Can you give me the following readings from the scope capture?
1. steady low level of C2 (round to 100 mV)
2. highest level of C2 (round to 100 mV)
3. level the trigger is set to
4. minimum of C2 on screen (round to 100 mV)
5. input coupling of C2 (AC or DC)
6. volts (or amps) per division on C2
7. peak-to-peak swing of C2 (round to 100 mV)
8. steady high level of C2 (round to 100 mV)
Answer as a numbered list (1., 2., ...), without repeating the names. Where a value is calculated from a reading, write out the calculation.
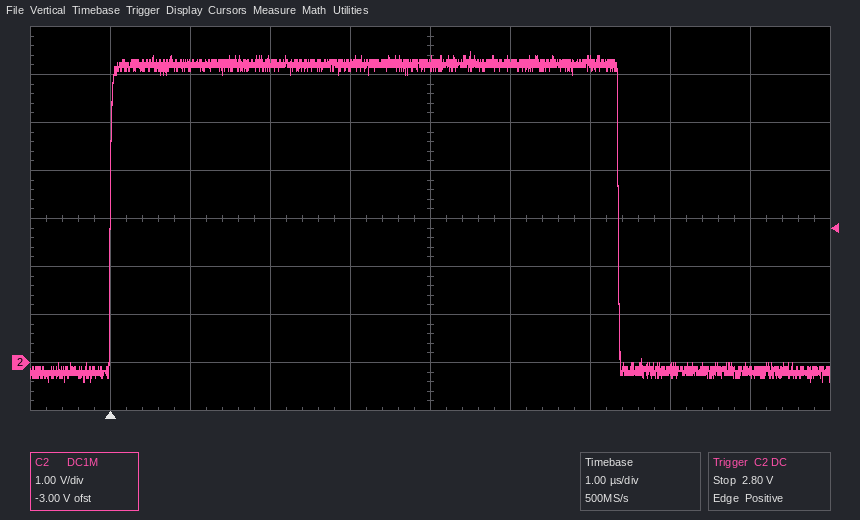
1. -200 mV
2. 6.5 V
3. 2.80 V
4. -400 mV
5. DC
6. 1 V
7. 6.5 V − (-400 mV) = 6.9 V
8. 6.2 V
